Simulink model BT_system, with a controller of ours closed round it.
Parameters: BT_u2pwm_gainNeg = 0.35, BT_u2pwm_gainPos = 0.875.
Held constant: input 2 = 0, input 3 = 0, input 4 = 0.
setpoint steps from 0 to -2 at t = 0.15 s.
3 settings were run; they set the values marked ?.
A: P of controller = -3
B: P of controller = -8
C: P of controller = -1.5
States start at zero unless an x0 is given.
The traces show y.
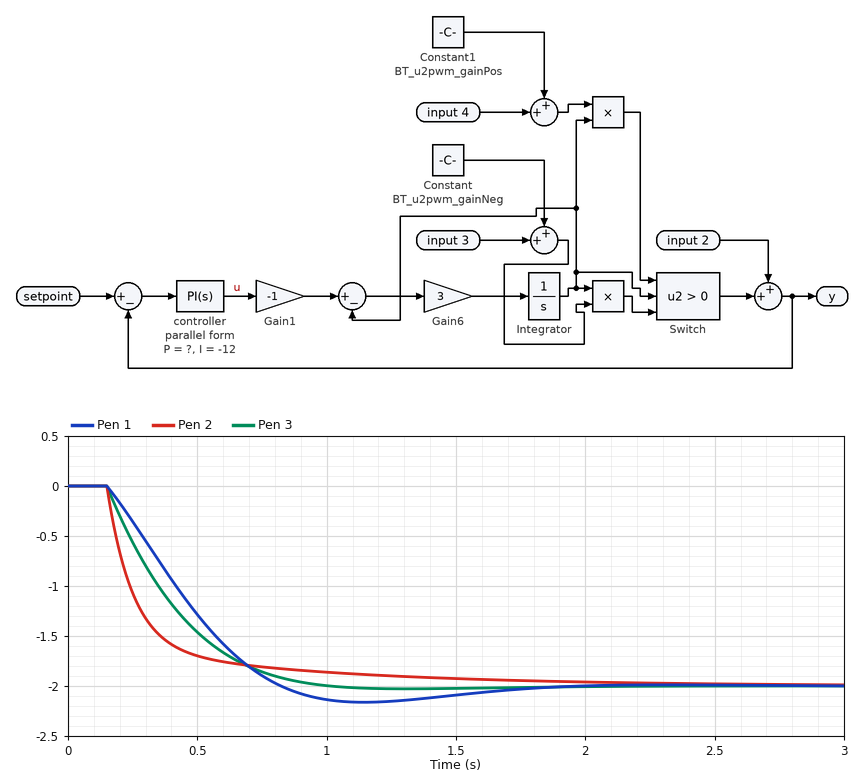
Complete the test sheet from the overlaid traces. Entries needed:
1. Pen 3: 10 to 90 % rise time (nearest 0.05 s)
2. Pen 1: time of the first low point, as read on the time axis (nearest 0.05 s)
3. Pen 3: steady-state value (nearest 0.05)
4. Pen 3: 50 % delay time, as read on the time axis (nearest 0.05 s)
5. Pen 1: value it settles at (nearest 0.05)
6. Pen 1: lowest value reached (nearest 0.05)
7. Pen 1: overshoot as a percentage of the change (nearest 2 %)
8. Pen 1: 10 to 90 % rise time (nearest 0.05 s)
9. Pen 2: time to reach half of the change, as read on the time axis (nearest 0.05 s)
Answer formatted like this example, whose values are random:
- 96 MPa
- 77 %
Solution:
- 0.50 s
- 1.15 s
- -2.00
- 0.35 s
- -2.00
- -2.15
- 8 %
- 0.50 s
- 0.25 s
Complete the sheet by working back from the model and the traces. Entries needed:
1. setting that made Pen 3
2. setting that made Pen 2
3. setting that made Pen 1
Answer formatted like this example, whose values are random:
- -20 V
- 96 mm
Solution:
- A
- B
- C
